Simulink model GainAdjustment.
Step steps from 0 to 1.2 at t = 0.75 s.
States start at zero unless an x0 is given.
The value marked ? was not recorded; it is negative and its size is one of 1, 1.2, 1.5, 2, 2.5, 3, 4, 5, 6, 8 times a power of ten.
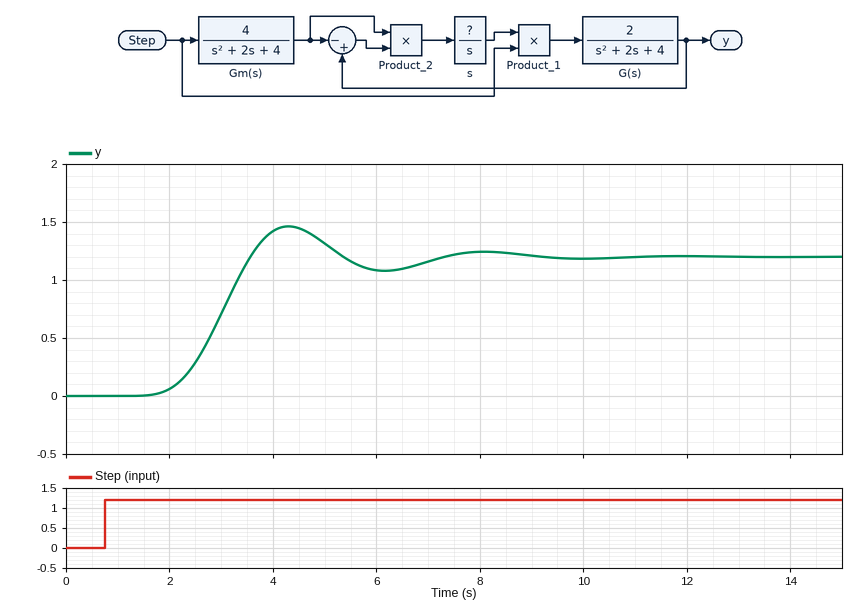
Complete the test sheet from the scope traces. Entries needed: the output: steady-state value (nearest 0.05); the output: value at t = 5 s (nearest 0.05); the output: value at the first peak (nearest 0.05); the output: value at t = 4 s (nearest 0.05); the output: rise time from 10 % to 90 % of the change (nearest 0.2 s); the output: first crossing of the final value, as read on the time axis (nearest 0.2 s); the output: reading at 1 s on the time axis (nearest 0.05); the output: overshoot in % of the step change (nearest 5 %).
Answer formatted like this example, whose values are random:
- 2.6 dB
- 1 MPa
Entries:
- 1.20
- 1.30
- 1.45
- 1.40
- 1.2 s
- 3.6 s
- 0.00
- 20 %
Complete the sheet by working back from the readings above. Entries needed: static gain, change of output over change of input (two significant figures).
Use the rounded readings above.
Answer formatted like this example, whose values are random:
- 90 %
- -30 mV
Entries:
- 1.0
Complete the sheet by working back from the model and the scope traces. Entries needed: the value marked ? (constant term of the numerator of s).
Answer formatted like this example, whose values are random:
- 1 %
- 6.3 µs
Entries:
- -1
